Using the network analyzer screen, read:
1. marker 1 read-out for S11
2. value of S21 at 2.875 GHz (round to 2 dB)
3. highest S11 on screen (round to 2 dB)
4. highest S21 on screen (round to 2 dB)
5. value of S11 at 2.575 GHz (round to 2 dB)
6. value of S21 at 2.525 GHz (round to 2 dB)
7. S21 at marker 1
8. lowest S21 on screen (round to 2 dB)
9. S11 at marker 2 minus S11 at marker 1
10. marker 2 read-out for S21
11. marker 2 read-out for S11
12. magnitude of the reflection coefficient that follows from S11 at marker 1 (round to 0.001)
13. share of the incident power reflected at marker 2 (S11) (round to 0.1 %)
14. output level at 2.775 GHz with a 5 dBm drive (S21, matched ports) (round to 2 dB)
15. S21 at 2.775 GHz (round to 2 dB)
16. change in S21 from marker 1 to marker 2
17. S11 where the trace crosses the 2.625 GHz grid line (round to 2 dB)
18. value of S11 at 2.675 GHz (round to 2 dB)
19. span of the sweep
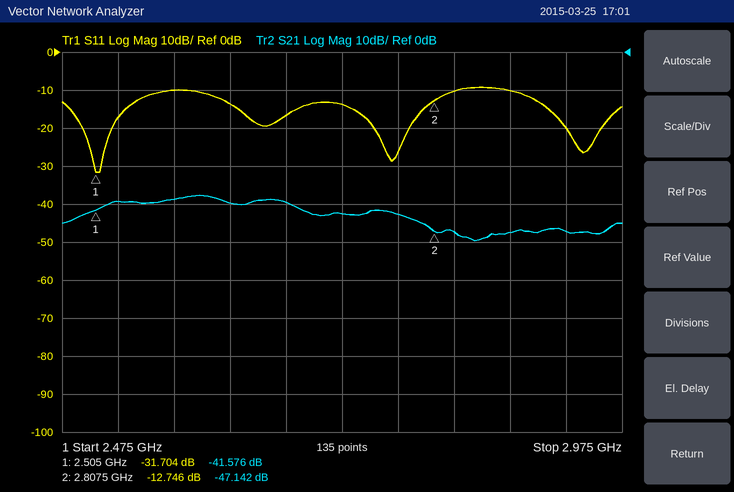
-31.704 dB
-48 dB
-10 dB
-38 dB
-10 dB
-40 dB
-41.576 dB
-50 dB
18.958 dB
-47.142 dB
-12.746 dB
0.026
5.3 %
-38 dBm
-42 dB
-5.566 dB
-14 dB
-16 dB
500 MHz
